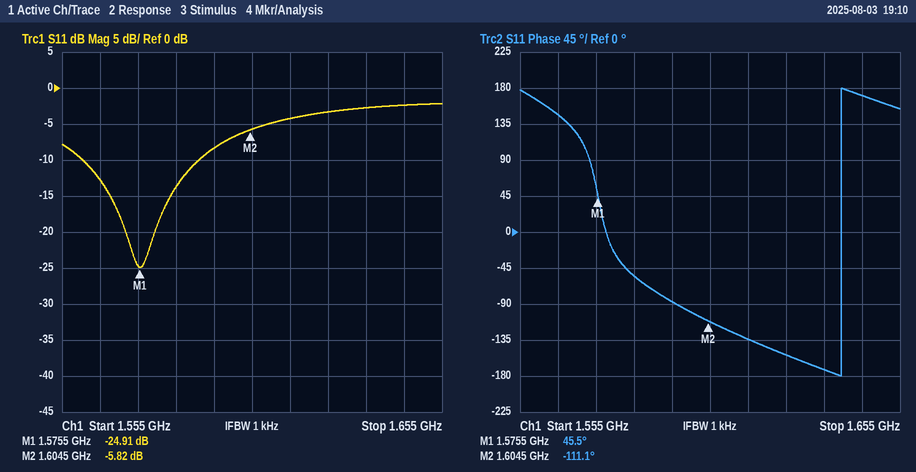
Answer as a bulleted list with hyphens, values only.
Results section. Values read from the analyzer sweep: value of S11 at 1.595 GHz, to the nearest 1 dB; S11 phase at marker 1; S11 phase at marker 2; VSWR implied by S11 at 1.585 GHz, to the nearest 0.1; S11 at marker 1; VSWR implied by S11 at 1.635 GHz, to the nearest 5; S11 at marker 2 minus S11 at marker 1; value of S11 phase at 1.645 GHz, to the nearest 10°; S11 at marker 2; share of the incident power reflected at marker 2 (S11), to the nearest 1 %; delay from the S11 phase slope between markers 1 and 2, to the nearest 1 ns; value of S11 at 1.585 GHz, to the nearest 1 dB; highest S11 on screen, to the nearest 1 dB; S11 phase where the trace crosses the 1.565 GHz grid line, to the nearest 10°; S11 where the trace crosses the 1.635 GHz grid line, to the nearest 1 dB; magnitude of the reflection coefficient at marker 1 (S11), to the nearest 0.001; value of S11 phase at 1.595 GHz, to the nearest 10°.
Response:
- -8 dB
- 45.5°
- -111.1°
- 1.5
- -24.91 dB
- 5
- 19.09 dB
- 170°
- -5.82 dB
- 26 %
- 15 ns
- -14 dB
- -2 dB
- 150°
- -3 dB
- 0.057
- -90°
